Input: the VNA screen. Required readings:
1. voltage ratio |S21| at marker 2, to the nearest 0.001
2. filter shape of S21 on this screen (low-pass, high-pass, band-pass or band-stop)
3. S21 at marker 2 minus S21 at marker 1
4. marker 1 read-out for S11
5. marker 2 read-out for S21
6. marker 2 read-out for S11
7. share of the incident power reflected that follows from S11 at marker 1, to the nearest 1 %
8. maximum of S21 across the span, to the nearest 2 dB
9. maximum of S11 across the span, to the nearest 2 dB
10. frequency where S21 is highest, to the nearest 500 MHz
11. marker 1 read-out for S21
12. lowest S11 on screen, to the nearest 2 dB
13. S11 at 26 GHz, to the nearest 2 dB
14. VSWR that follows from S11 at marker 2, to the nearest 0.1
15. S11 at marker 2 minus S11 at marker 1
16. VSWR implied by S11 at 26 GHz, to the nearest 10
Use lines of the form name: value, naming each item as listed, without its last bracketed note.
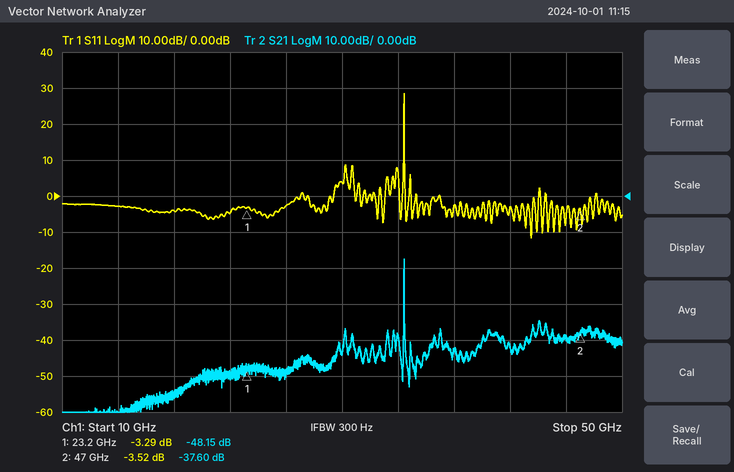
voltage ratio |S21| at marker 2, to the nearest 0.001: 0.013
filter shape of S21 on this screen: band-pass
S21 at marker 2 minus S21 at marker 1: 10.55 dB
marker 1 read-out for S11: -3.29 dB
marker 2 read-out for S21: -37.60 dB
marker 2 read-out for S11: -3.52 dB
share of the incident power reflected that follows from S11 at marker 1, to the nearest 1 %: 47 %
maximum of S21 across the span, to the nearest 2 dB: -18 dB
maximum of S11 across the span, to the nearest 2 dB: 28 dB
frequency where S21 is highest, to the nearest 500 MHz: 34.5 GHz
marker 1 read-out for S21: -48.15 dB
lowest S11 on screen, to the nearest 2 dB: -12 dB
S11 at 26 GHz, to the nearest 2 dB: -2 dB
VSWR that follows from S11 at marker 2, to the nearest 0.1: 5.0
S11 at marker 2 minus S11 at marker 1: -0.23 dB
VSWR implied by S11 at 26 GHz, to the nearest 10: 10
